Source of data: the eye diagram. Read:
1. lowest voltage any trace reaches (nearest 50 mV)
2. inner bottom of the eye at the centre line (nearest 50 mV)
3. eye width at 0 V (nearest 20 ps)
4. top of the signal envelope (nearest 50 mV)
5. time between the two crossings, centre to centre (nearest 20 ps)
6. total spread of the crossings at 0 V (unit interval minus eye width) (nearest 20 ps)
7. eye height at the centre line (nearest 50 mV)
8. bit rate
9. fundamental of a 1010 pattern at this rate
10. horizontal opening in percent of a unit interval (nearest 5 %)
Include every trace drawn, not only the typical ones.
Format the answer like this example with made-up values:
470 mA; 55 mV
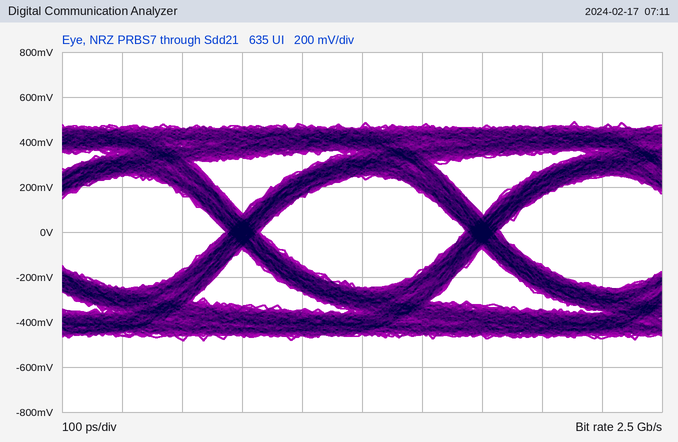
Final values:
-500 mV; -250 mV; 340 ps; 500 mV; 400 ps; 60 ps; 500 mV; 2.5 Gb/s; 1.25 GHz; 85 %
